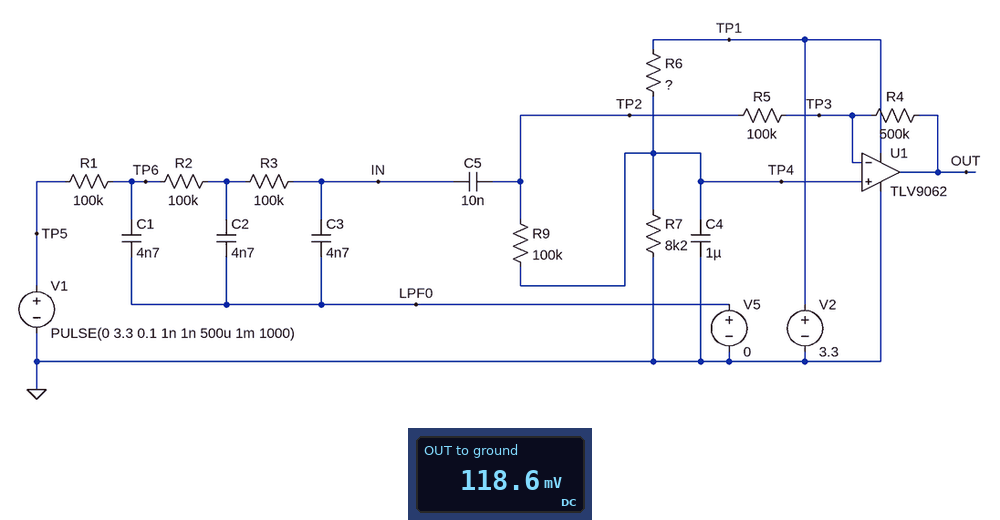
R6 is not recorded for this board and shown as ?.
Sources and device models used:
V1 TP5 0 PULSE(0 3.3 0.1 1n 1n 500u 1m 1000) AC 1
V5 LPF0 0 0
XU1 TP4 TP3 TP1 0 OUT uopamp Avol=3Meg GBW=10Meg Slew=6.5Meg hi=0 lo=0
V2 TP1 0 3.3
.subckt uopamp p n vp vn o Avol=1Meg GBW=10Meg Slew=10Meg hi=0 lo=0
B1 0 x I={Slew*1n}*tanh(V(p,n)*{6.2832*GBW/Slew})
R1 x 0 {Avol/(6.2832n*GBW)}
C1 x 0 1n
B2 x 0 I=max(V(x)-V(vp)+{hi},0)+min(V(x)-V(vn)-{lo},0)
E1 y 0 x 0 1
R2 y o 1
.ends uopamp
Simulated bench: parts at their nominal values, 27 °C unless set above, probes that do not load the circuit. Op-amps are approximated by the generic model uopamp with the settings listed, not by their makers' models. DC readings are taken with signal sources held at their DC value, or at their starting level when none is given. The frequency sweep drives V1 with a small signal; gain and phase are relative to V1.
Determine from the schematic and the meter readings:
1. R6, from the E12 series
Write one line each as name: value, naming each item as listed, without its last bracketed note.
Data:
R6, from the E12 series: 220 kΩ
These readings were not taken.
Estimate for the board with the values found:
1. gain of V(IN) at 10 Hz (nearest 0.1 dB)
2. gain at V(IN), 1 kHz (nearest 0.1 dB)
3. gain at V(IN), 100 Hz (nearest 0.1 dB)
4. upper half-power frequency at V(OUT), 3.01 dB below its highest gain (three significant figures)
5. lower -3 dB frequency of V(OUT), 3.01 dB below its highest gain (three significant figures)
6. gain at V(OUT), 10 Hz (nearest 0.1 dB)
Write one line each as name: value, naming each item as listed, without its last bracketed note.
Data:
gain of V(IN) at 10 Hz: -0.5 dB
gain at V(IN), 1 kHz: -35.7 dB
gain at V(IN), 100 Hz: -11.2 dB
upper half-power frequency at V(OUT), 3.01 dB below its highest gain: 333 Hz
lower -3 dB frequency of V(OUT), 3.01 dB below its highest gain: 24.7 Hz
gain at V(OUT), 10 Hz: -16.7 dB
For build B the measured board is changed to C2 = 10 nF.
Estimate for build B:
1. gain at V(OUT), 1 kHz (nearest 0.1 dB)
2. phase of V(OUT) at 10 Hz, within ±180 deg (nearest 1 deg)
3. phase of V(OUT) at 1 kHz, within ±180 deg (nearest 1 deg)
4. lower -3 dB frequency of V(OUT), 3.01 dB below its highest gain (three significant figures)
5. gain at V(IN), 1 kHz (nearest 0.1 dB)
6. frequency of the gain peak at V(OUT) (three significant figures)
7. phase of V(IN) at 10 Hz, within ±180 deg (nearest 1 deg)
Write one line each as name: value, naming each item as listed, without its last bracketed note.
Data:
gain at V(OUT), 1 kHz: -27.4 dB
phase of V(OUT) at 10 Hz, within ±180 deg: -115 deg
phase of V(OUT) at 1 kHz, within ±180 deg: 15 deg
lower -3 dB frequency of V(OUT), 3.01 dB below its highest gain: 20.9 Hz
gain at V(IN), 1 kHz: -40.9 dB
frequency of the gain peak at V(OUT): 73.9 Hz
phase of V(IN) at 10 Hz, within ±180 deg: -24 deg
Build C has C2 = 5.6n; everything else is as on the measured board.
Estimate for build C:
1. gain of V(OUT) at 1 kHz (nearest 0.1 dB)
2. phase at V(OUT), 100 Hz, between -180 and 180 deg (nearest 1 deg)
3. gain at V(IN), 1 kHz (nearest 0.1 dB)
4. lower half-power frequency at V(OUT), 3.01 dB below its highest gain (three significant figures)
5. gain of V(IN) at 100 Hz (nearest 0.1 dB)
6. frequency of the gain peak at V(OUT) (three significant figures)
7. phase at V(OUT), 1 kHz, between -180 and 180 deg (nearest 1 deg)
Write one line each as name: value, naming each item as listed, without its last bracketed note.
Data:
gain of V(OUT) at 1 kHz: -23.2 dB
phase at V(OUT), 100 Hz, between -180 and 180 deg: 167 deg
gain at V(IN), 1 kHz: -36.8 dB
lower half-power frequency at V(OUT), 3.01 dB below its highest gain: 23.9 Hz
gain of V(IN) at 100 Hz: -11.5 dB
frequency of the gain peak at V(OUT): 89.4 Hz
phase at V(OUT), 1 kHz, between -180 and 180 deg: 24 deg
